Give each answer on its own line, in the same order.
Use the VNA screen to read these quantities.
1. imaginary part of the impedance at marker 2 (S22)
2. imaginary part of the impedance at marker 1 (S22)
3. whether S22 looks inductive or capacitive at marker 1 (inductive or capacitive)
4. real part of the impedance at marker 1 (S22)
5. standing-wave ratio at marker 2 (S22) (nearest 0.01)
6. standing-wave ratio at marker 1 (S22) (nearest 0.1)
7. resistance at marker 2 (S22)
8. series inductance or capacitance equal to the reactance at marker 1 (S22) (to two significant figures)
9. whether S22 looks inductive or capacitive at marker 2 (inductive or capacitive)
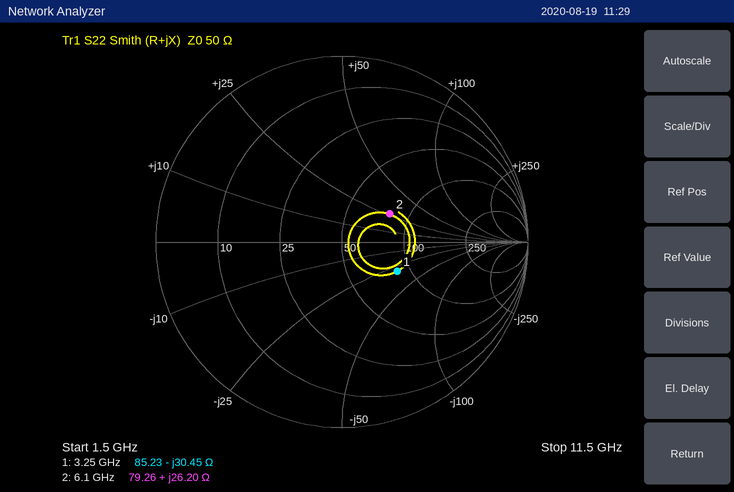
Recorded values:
+26.20 Ω
-30.45 Ω
capacitive
85.23 Ω
1.85
2.0
79.26 Ω
1.6 pF
inductive
